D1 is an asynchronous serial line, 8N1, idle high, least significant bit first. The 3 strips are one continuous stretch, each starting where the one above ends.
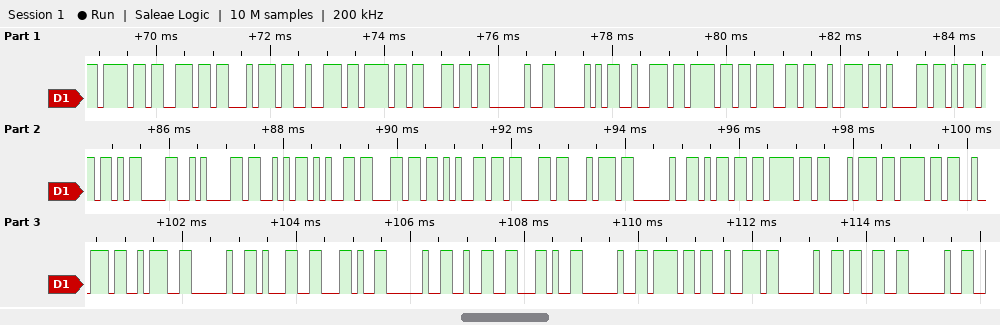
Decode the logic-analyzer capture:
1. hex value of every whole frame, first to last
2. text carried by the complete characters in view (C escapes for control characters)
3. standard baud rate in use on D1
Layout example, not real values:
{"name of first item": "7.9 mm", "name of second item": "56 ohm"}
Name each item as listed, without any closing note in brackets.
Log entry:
{"hex value of every whole frame, first to last": "6F 6E 74 72 6F 6C 20 50 72 6F 67 72 61 6D 0D 0A 53 65 6C 65 63 74 20 6D 6F 74 6F 72 3A 20 31 2C 20 32 2C 20 6F 72 20 33 20", "text carried by the complete characters in view": "\"ontrol Program\\r\\nSelect motor: 1, 2, or 3 \"", "standard baud rate in use on D1": "9600 baud"}
